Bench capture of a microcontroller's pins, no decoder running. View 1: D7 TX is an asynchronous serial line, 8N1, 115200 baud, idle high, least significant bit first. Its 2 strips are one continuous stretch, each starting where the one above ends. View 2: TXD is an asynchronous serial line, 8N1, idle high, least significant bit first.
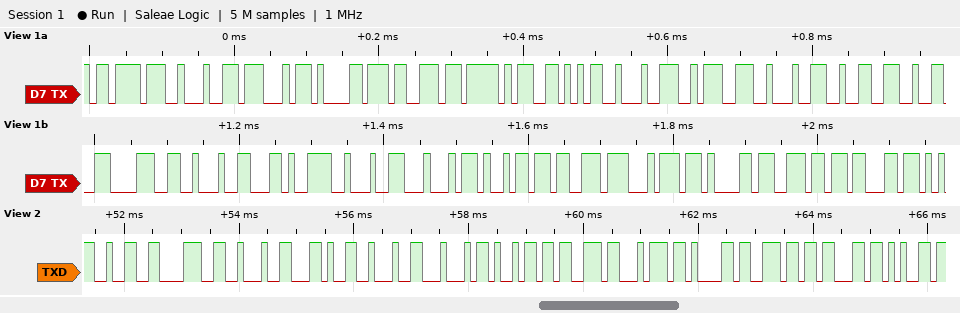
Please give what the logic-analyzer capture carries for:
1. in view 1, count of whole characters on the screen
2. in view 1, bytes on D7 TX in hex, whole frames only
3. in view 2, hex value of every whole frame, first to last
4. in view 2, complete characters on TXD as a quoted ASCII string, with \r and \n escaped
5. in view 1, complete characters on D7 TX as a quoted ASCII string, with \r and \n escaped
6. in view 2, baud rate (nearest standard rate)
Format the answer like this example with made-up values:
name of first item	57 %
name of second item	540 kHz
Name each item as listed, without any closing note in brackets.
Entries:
in view 1, count of whole characters on the screen	23
in view 1, bytes on D7 TX in hex, whole frames only	7B 22 47 61 73 5F 56 22 3A 22 32 32 38 22 2C 22 44 69 73 74 61 6E 63
in view 2, hex value of every whole frame, first to last	0x32 0x38 0x22 0x2C 0x22 0x44 0x69 0x73 0x74 0x61 0x6E 0x63 0x65
in view 2, complete characters on TXD as a quoted ASCII string, with \r and \n escaped	"28\",\"Distance"
in view 1, complete characters on D7 TX as a quoted ASCII string, with \r and \n escaped	"{\"Gas_V\":\"228\",\"Distanc"
in view 2, baud rate	9600 baud
